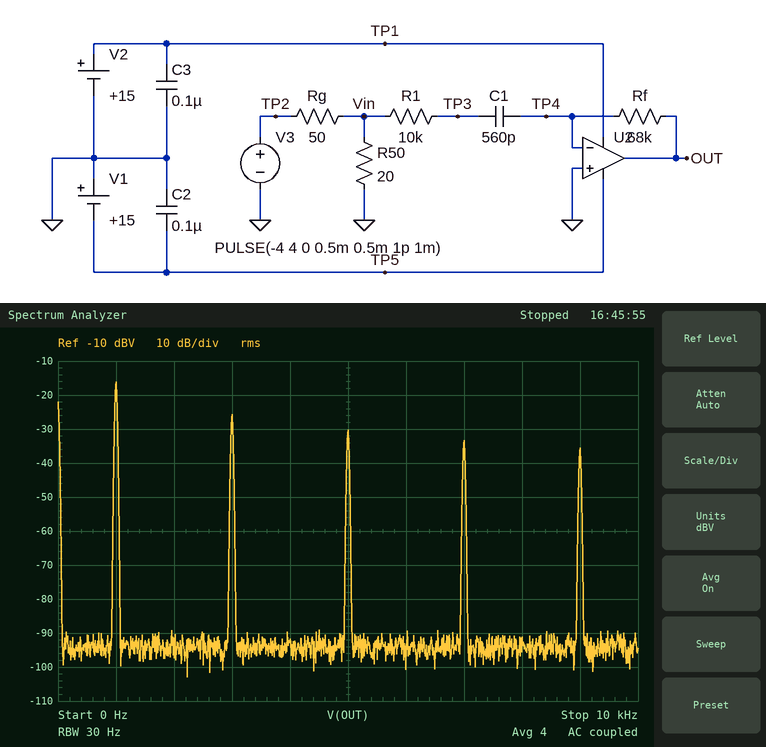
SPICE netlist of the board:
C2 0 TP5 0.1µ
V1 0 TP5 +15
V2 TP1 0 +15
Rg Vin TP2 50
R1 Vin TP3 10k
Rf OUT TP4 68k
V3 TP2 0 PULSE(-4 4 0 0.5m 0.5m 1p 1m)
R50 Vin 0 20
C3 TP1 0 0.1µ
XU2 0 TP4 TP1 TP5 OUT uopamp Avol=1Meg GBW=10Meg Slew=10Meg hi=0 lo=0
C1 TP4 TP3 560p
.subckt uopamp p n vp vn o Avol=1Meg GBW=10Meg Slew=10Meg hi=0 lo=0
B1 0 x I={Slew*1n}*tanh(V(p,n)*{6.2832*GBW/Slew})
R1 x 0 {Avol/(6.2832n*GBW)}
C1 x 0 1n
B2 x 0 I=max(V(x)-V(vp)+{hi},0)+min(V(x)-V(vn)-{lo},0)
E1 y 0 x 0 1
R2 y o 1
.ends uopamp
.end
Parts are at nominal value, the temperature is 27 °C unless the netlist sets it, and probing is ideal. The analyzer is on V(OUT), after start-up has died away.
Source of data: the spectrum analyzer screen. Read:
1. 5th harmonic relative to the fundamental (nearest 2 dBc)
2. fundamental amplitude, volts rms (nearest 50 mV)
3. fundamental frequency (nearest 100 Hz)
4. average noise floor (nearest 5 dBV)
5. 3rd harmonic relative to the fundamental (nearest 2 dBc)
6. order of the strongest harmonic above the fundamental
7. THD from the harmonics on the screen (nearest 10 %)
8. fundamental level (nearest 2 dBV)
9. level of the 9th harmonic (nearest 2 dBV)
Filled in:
-14 dBc
150 mV
1.0 kHz
-95 dBV
-10 dBc
3
40 %
-16 dBV
-36 dBV
